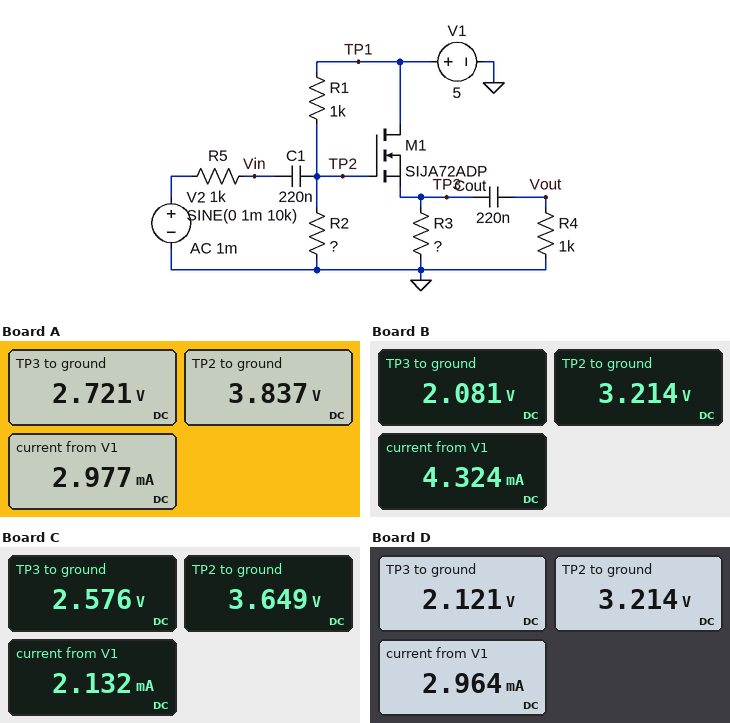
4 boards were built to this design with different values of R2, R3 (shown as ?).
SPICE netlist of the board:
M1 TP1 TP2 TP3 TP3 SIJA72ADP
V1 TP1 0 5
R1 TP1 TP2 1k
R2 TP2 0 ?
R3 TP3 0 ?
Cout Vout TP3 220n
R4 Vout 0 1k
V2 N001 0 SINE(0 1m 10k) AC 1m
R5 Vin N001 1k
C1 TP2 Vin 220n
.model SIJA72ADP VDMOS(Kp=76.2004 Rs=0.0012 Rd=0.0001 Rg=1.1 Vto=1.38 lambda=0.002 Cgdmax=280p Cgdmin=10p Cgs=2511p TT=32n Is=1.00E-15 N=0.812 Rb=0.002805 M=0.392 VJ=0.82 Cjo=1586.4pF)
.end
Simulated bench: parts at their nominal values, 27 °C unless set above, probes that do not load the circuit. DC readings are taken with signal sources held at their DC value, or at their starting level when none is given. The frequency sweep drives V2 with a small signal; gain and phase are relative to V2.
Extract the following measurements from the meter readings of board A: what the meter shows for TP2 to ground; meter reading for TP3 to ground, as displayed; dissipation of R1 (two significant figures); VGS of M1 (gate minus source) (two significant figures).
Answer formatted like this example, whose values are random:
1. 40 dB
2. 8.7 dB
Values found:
1. 3.837 V
2. 2.721 V
3. 1.4 mW
4. 1.1 V
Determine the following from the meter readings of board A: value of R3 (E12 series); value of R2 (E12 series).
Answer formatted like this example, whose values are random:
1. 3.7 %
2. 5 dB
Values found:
1. 1.5 kΩ
2. 3.3 kΩ
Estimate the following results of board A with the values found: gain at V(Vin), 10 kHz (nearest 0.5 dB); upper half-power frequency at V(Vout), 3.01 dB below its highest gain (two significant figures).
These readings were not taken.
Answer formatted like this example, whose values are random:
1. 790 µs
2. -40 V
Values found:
1. -7.0 dB
2. 1.1 MHz
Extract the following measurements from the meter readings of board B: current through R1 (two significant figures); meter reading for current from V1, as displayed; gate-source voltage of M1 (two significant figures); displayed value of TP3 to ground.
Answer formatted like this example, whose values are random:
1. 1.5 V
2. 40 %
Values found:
1. 1.8 mA
2. 4.324 mA
3. 1.1 V
4. 2.081 V
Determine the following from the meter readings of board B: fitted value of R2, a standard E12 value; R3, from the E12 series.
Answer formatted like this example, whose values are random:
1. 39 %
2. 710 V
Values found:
1. 1.8 kΩ
2. 820 Ω
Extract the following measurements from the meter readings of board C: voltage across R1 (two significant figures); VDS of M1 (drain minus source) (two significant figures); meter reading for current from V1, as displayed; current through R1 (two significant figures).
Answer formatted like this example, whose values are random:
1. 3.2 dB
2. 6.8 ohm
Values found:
1. 1.4 V
2. 2.4 V
3. 2.132 mA
4. 1.4 mA
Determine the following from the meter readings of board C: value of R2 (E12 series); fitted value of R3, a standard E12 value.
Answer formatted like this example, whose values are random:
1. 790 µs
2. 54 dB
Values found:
1. 2.7 kΩ
2. 3.3 kΩ
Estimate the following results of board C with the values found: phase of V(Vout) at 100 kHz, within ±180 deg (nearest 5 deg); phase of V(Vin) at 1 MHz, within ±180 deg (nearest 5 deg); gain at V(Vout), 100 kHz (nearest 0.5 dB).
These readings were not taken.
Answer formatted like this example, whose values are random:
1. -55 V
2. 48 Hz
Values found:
1. -5 deg
2. -75 deg
3. -8.0 dB
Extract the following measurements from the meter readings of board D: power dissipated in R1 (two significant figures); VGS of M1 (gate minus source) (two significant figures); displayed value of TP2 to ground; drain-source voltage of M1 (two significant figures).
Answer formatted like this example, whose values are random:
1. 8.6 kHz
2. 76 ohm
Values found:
1. 3.2 mW
2. 1.1 V
3. 3.214 V
4. 2.9 V
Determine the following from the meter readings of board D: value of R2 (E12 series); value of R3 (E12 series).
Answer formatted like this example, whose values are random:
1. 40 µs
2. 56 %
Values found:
1. 1.8 kΩ
2. 1.8 kΩ
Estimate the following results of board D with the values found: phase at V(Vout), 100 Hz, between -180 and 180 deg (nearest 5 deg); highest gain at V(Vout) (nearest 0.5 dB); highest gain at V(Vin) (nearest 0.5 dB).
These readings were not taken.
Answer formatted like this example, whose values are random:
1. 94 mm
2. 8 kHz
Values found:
1. 160 deg
2. -7.5 dB
3. 0 dB
